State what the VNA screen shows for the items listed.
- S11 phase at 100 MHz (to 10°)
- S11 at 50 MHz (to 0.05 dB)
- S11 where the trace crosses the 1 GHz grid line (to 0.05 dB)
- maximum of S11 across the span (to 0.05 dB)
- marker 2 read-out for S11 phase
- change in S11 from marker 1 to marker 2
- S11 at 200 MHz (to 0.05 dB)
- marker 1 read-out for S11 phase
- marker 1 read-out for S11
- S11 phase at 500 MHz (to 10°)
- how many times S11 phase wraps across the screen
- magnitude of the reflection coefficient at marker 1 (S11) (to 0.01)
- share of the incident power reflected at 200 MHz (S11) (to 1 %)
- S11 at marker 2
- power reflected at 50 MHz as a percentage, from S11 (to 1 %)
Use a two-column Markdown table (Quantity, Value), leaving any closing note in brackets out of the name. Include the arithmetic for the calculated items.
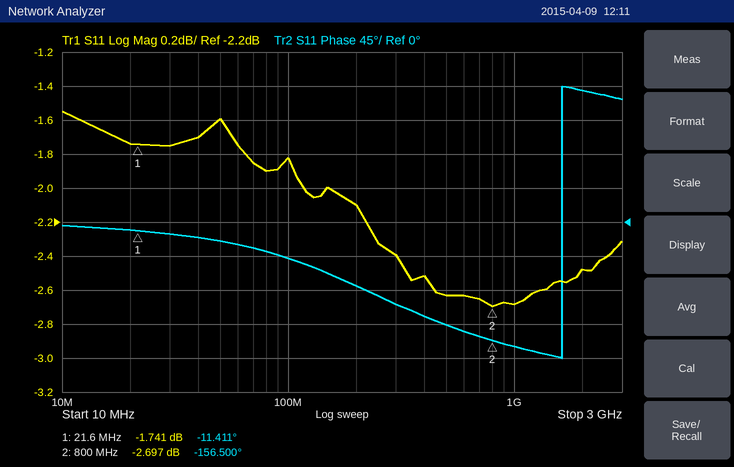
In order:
| Quantity | Value |
|---|---|
| S11 phase at 100 MHz | -50° |
| S11 at 50 MHz | -1.60 dB |
| S11 where the trace crosses the 1 GHz grid line | -2.70 dB |
| maximum of S11 across the span | -1.55 dB |
| marker 2 read-out for S11 phase | -156.500° |
| change in S11 from marker 1 to marker 2 | -2.697 − (-1.741) = -0.956 dB |
| S11 at 200 MHz | -2.10 dB |
| marker 1 read-out for S11 phase | -11.411° |
| marker 1 read-out for S11 | -1.741 dB |
| S11 phase at 500 MHz | -140° |
| how many times S11 phase wraps across the screen | 1 |
| magnitude of the reflection coefficient at marker 1 (S11) | 10^(-1.741/20) ≈ 0.82 |
| share of the incident power reflected at 200 MHz (S11) | 10^(-2.1/10) ≈ 62 % |
| S11 at marker 2 | -2.697 dB |
| power reflected at 50 MHz as a percentage, from S11 | 10^(-1.6/10) ≈ 69 % |
